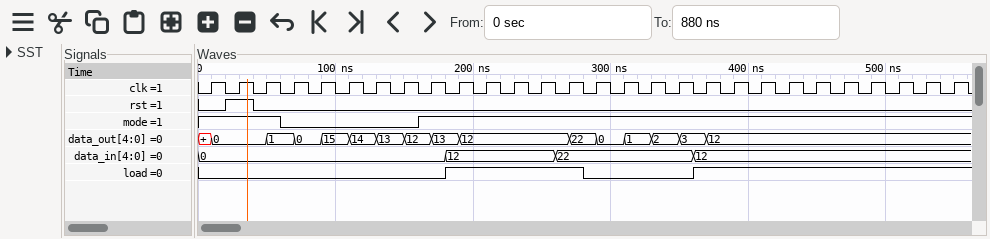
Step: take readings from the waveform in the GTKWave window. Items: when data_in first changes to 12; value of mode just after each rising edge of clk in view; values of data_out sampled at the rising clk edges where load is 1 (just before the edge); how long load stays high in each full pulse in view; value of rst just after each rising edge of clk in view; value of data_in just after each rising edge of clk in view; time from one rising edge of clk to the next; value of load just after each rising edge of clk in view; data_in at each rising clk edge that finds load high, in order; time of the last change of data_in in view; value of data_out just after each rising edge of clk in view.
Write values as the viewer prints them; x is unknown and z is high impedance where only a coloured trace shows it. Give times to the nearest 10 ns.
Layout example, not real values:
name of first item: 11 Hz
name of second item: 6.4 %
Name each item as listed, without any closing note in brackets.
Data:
when data_in first changes to 12: 180 ns
value of mode just after each rising edge of clk in view: 1 1 1 0 0 0 0 0 1 1 1 1 1 1 1 1 1 1 1 1 1 1 1 1 1 1 1 1
values of data_out sampled at the rising clk edges where load is 1: 13, 12, 12, 12, 12, 3, 12, 12, 12, 12, 12, 12, 12, 12, 12
how long load stays high in each full pulse in view: 100 ns
value of rst just after each rising edge of clk in view: 0 1 0 0 0 0 0 0 0 0 0 0 0 0 0 0 0 0 0 0 0 0 0 0 0 0 0 0
value of data_in just after each rising edge of clk in view: 0, 0, 0, 0, 0, 0, 0, 0, 0, 12, 12, 12, 12, 22, 22, 22, 22, 22, 12, 12, 12, 12, 12, 12, 12, 12, 12, 12
time from one rising edge of clk to the next: 20 ns
value of load just after each rising edge of clk in view: 0 0 0 0 0 0 0 0 0 1 1 1 1 1 0 0 0 0 1 1 1 1 1 1 1 1 1 1
data_in at each rising clk edge that finds load high, in order: 12, 12, 12, 12, 22, 12, 12, 12, 12, 12, 12, 12, 12, 12, 12
time of the last change of data_in in view: 360 ns
value of data_out just after each rising edge of clk in view: 0, 0, 1, 0, 15, 14, 13, 12, 13, 12, 12, 12, 12, 22, 0, 1, 2, 3, 12, 12, 12, 12, 12, 12, 12, 12, 12, 12
